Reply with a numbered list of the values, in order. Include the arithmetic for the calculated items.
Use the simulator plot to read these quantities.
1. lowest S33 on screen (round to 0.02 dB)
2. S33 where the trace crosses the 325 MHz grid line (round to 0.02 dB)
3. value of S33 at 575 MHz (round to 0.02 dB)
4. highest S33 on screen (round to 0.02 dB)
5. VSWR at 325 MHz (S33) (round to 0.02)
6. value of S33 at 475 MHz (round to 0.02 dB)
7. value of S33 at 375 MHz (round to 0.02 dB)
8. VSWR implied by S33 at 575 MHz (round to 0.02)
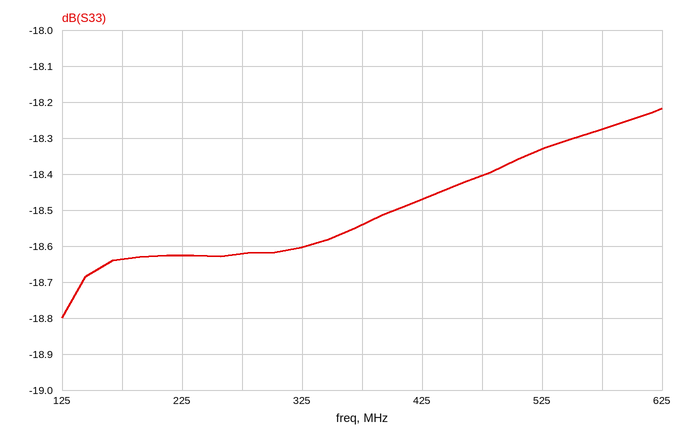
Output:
1. -18.80 dB
2. -18.60 dB
3. -18.28 dB
4. -18.22 dB
5. |Γ| = 10^(-18.6/20) = 0.1175; VSWR = (1 + 0.1175)/(1 − 0.1175) ≈ 1.27, so 1.26 to the nearest 0.02
6. -18.40 dB
7. -18.54 dB
8. |Γ| = 10^(-18.28/20) = 0.1219; VSWR = (1 + 0.1219)/(1 − 0.1219) ≈ 1.28
